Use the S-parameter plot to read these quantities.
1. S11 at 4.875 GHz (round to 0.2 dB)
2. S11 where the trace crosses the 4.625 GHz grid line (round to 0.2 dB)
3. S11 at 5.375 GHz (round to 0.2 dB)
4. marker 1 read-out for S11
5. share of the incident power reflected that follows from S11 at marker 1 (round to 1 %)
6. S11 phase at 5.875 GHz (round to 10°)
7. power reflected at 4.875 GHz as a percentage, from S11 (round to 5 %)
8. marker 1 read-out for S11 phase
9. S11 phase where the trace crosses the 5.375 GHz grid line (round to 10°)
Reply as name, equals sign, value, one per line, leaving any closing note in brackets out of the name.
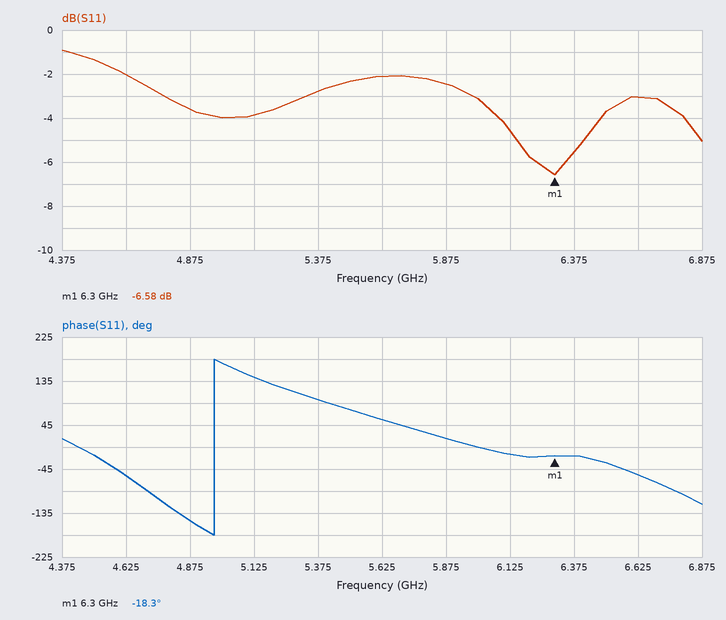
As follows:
S11 at 4.875 GHz = -3.6 dB
S11 where the trace crosses the 4.625 GHz grid line = -2.0 dB
S11 at 5.375 GHz = -2.8 dB
marker 1 read-out for S11 = -6.58 dB
share of the incident power reflected that follows from S11 at marker 1 = 22 %
S11 phase at 5.875 GHz = 20°
power reflected at 4.875 GHz as a percentage, from S11 = 45 %
marker 1 read-out for S11 phase = -18.3°
S11 phase where the trace crosses the 5.375 GHz grid line = 100°
